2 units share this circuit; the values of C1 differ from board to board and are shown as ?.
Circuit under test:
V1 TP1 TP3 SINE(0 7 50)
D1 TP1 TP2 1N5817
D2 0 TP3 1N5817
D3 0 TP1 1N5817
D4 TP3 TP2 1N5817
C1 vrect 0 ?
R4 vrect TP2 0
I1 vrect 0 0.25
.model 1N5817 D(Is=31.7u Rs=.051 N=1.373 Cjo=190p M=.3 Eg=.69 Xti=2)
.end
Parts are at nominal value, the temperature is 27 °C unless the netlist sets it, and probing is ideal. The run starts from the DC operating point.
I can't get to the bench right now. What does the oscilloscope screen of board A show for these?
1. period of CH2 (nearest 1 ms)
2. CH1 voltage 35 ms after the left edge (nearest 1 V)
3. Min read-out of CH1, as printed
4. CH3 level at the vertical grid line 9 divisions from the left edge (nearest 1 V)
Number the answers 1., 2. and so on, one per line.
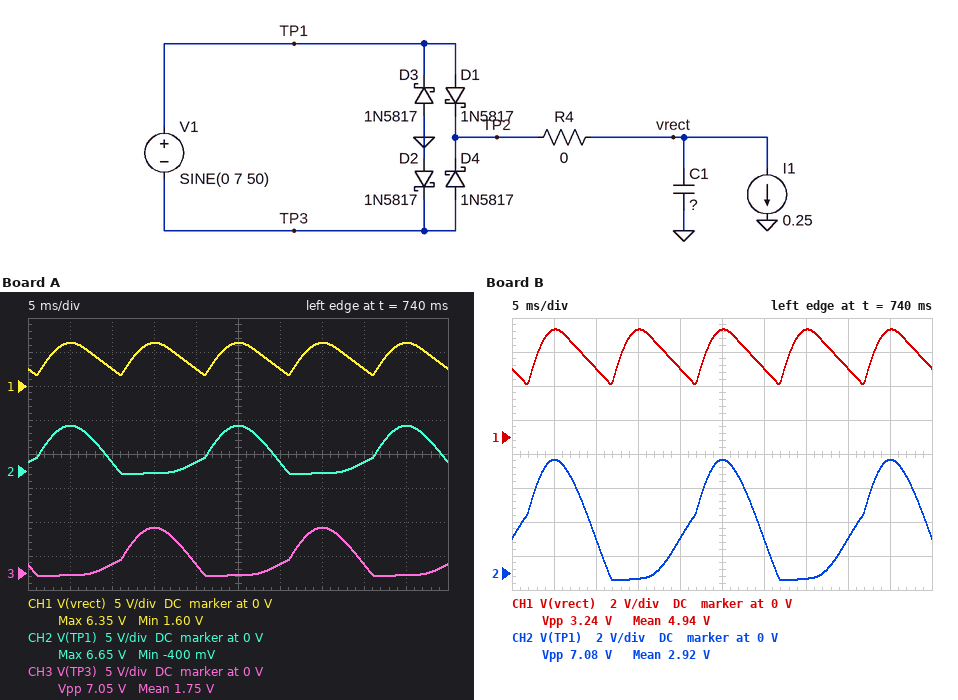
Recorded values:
1. 20 ms
2. 6 V
3. 1.60 V
4. 0 V
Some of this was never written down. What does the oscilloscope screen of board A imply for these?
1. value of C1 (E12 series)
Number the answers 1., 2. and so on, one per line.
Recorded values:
1. 270 µF
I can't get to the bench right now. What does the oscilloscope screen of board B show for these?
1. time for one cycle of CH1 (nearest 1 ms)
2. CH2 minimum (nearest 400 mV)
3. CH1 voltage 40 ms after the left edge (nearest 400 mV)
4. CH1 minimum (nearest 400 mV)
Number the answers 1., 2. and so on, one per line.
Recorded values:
1. 10 ms
2. -400 mV
3. 4.0 V
4. 3.2 V
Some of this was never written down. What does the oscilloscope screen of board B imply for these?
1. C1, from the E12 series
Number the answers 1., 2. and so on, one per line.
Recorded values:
1. 470 µF
